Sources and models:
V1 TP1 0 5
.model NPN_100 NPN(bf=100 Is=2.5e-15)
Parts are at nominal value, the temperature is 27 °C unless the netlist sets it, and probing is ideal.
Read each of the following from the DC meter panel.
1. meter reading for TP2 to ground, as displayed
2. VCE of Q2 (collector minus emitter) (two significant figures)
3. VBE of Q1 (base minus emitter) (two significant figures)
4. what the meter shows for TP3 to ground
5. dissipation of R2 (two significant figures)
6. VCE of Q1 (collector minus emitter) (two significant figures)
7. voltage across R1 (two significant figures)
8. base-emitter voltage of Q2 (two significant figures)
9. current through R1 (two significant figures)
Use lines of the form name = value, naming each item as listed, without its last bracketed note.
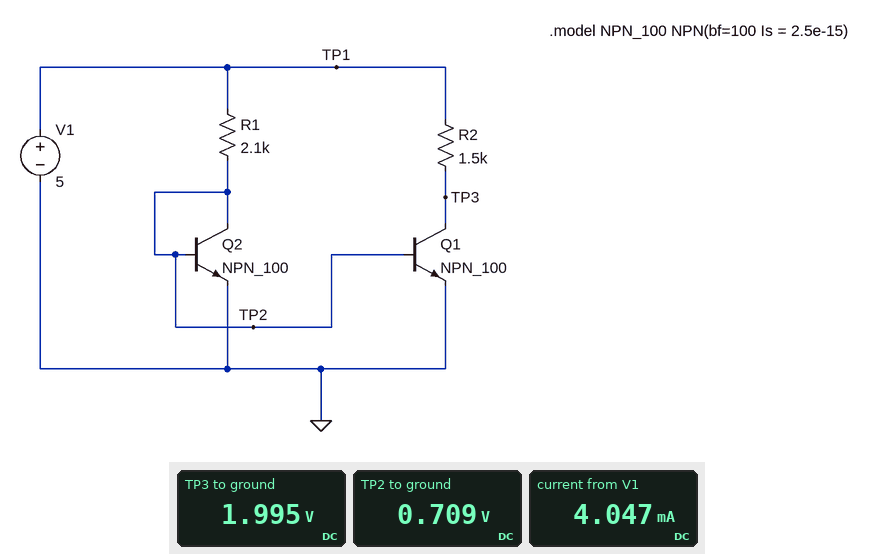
meter reading for TP2 to ground, as displayed = 0.709 V
VCE of Q2 (collector minus emitter) = 710 mV
VBE of Q1 (base minus emitter) = 710 mV
what the meter shows for TP3 to ground = 1.995 V
dissipation of R2 = 6.0 mW
VCE of Q1 (collector minus emitter) = 2.0 V
voltage across R1 = 4.3 V
base-emitter voltage of Q2 = 710 mV
current through R1 = 2.0 mA
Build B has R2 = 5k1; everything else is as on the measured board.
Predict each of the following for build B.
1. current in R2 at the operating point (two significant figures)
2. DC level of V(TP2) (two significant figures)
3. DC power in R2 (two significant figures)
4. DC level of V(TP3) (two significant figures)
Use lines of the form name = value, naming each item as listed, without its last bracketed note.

current in R2 at the operating point = 970 µA
DC level of V(TP2) = 700 mV
DC power in R2 = 4.8 mW
DC level of V(TP3) = 41 mV
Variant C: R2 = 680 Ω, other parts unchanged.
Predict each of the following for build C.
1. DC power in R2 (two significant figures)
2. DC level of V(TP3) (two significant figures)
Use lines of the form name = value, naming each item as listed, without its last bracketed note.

DC power in R2 = 2.7 mW
DC level of V(TP3) = 3.6 V
